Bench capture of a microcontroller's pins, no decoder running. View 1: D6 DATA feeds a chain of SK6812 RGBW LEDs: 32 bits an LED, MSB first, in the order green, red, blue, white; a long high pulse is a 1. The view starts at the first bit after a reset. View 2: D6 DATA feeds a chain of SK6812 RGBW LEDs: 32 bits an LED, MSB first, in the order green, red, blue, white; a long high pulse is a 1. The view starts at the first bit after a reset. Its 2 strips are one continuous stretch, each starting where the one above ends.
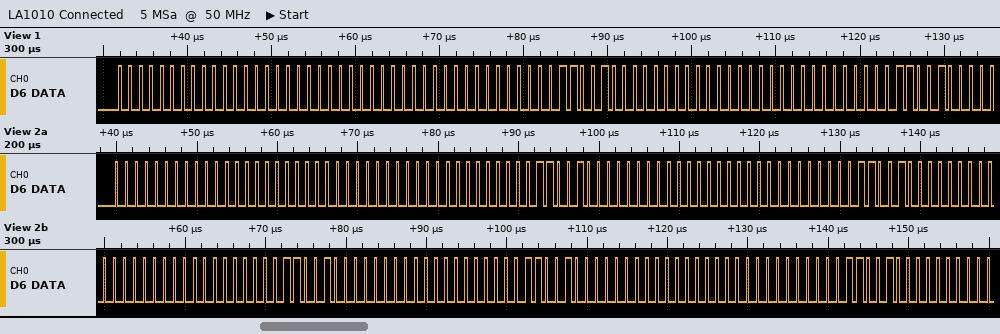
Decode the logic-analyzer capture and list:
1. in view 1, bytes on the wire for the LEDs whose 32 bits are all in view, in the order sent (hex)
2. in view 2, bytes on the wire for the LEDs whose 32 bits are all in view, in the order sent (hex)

00 00 00 00 00 32 00 00
00 00 00 00 00 32 00 00 00 32 00 00 00 32 00 00 32 00 00 00
